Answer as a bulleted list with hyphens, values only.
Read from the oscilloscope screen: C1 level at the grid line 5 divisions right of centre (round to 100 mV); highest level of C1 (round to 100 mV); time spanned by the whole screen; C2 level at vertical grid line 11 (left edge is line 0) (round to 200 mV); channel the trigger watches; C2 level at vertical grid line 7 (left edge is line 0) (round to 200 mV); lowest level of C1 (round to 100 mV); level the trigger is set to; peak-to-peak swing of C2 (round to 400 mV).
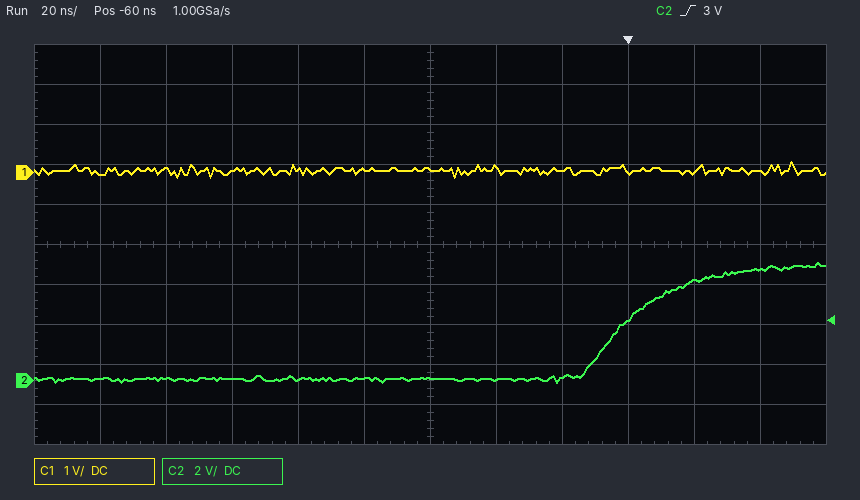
- 0.0 V
- 300 mV
- 240 ns
- 5.6 V
- C2
- 0.0 V
- -100 mV
- 3 V
- 6.0 V
